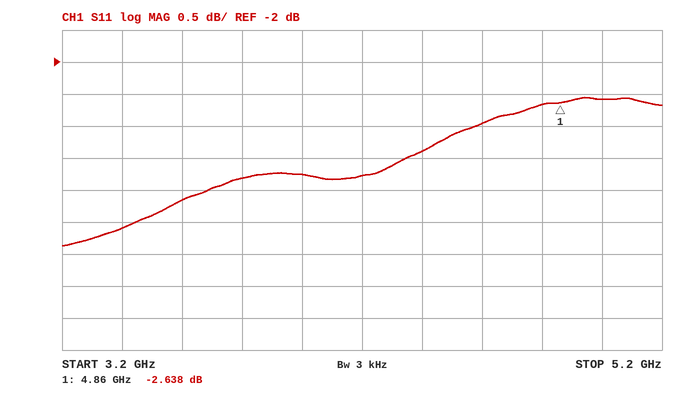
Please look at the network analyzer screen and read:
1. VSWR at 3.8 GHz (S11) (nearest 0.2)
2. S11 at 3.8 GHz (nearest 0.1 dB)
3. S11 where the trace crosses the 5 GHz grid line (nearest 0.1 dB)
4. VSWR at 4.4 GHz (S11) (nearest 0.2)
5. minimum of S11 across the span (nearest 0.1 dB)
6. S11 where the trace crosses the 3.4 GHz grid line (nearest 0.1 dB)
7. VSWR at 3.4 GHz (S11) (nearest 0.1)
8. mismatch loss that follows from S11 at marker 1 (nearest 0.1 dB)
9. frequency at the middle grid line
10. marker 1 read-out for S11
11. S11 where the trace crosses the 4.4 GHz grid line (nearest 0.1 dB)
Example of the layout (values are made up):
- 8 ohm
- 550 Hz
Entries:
- 4.6
- -3.8 dB
- -2.6 dB
- 5.2
- -4.9 dB
- -4.6 dB
- 3.9
- 3.4 dB
- 4.2 GHz
- -2.638 dB
- -3.4 dB
